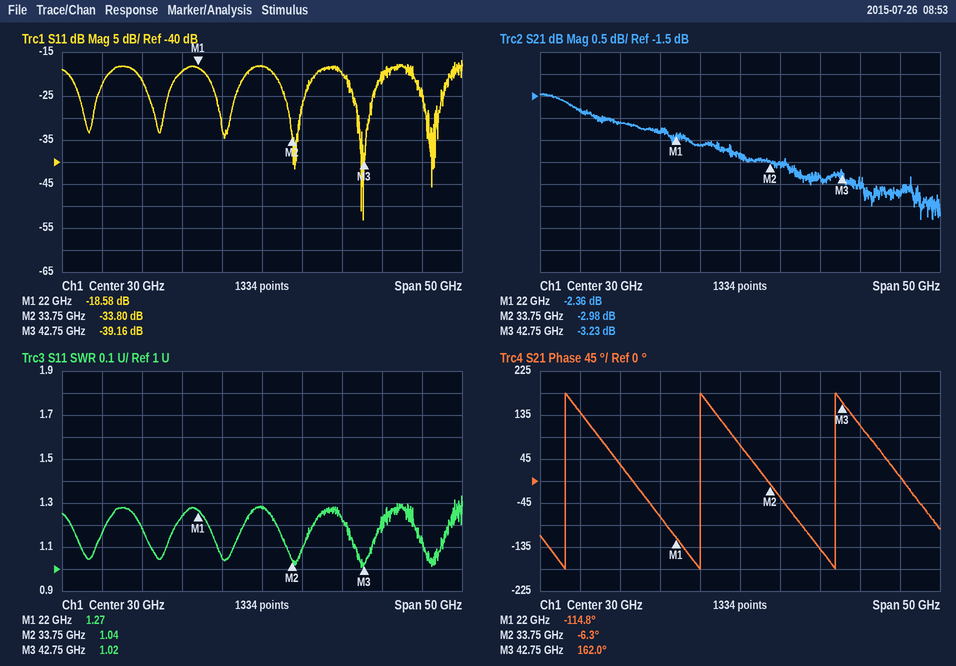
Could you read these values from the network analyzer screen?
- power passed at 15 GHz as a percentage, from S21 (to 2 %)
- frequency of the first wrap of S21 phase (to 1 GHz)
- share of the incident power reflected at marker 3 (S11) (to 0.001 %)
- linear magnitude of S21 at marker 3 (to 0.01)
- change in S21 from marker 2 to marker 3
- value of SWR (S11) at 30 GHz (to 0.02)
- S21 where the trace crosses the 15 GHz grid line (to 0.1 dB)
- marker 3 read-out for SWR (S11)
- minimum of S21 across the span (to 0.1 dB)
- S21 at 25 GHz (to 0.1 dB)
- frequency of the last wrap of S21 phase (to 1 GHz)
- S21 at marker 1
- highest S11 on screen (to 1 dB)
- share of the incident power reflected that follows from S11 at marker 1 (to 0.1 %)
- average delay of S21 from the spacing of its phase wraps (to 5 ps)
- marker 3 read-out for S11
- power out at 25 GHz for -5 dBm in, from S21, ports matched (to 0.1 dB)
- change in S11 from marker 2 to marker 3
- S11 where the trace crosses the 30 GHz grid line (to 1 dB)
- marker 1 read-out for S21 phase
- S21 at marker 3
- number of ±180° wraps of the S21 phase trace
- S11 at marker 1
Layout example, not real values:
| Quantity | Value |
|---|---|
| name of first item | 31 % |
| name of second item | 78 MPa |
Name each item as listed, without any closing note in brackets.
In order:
| Quantity | Value |
|---|---|
| power passed at 15 GHz as a percentage, from S21 | 62 % |
| frequency of the first wrap of S21 phase | 8 GHz |
| share of the incident power reflected at marker 3 (S11) | 0.012 % |
| linear magnitude of S21 at marker 3 | 0.69 |
| change in S21 from marker 2 to marker 3 | -0.25 dB |
| value of SWR (S11) at 30 GHz | 1.28 |
| S21 where the trace crosses the 15 GHz grid line | -2.1 dB |
| marker 3 read-out for SWR | 1.02 |
| minimum of S21 across the span | -4.3 dB |
| S21 at 25 GHz | -2.6 dB |
| frequency of the last wrap of S21 phase | 42 GHz |
| S21 at marker 1 | -2.36 dB |
| highest S11 on screen | -17 dB |
| share of the incident power reflected that follows from S11 at marker 1 | 1.4 % |
| average delay of S21 from the spacing of its phase wraps | 60 ps |
| marker 3 read-out for S11 | -39.16 dB |
| power out at 25 GHz for -5 dBm in, from S21, ports matched | -7.6 dBm |
| change in S11 from marker 2 to marker 3 | -5.36 dB |
| S11 where the trace crosses the 30 GHz grid line | -18 dB |
| marker 1 read-out for S21 phase | -114.8° |
| S21 at marker 3 | -3.23 dB |
| number of ±180° wraps of the S21 phase trace | 3 |
| S11 at marker 1 | -18.58 dB |
